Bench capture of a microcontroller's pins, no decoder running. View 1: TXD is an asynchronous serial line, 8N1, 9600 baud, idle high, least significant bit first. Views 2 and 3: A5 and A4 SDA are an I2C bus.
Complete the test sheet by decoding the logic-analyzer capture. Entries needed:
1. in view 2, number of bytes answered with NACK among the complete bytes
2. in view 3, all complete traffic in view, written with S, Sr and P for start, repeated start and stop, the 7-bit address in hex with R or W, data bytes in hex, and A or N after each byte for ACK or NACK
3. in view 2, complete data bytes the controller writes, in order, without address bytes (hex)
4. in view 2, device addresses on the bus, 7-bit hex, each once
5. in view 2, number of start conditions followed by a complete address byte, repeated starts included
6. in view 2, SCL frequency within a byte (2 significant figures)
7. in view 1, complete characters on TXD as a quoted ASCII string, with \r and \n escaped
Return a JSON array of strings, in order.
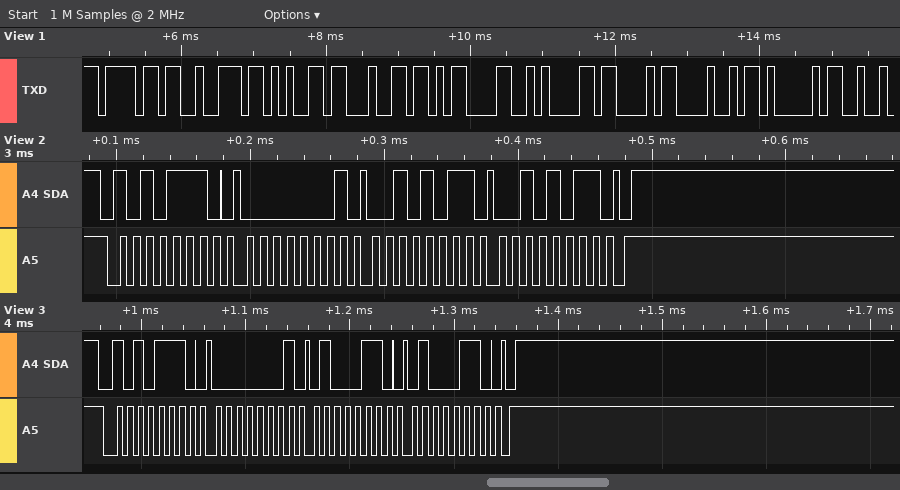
["0", "S 57W A 01 A 46 A 46 A P", "01 2B 2B", "0x57", "1", "100 kHz", "\"ored\\r\\nCHA\""]
